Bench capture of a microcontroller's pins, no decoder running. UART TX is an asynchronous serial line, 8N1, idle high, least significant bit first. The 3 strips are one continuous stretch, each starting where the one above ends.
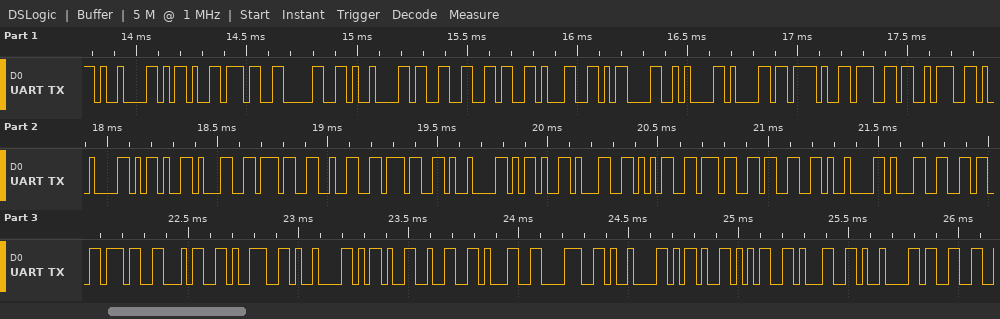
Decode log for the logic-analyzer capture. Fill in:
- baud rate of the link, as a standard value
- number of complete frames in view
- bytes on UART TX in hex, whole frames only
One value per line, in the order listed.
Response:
38400 baud
43
09 2D 37 30 09 33 36 31 0D 0A 61 2F 67 3A 09 2D 31 37 32 37 09 2D 31 35 37 33 09 31 36 37 34 39 09 2D 32 31 38 09 2D 35 31 09 33
